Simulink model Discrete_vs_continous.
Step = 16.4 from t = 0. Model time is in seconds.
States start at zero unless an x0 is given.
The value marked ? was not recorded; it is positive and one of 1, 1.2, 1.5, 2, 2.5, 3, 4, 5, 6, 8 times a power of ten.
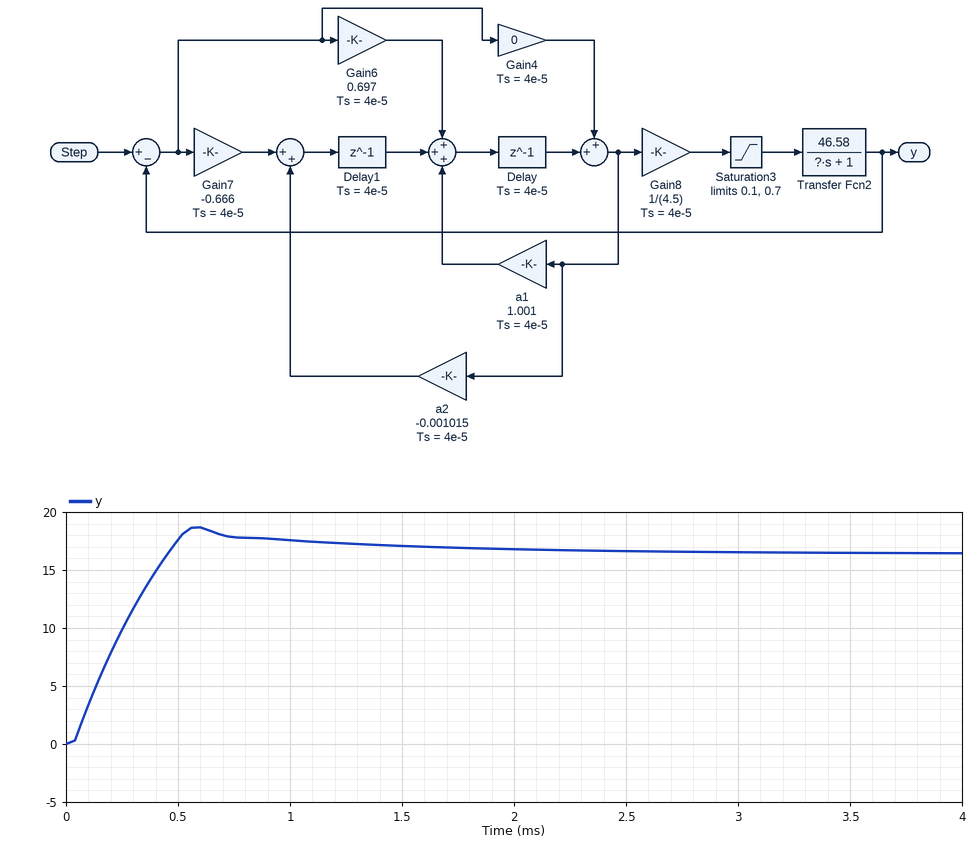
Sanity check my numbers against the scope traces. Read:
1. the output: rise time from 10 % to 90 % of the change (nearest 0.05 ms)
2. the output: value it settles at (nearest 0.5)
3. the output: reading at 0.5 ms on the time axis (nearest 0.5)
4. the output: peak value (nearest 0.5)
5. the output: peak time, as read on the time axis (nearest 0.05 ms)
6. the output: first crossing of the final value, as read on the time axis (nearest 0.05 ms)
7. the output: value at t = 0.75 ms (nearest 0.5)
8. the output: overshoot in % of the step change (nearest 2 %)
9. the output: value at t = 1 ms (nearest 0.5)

0.35 ms
16.5
17.5
18.5
0.60 ms
0.45 ms
18.0
14 %
17.5
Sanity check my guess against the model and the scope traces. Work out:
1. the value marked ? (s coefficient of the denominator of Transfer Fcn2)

0.0006
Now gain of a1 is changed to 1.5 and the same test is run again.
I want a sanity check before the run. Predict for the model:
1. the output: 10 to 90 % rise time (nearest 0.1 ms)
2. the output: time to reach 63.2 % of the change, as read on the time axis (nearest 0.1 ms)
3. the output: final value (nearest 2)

1.3 ms
0.6 ms
32
